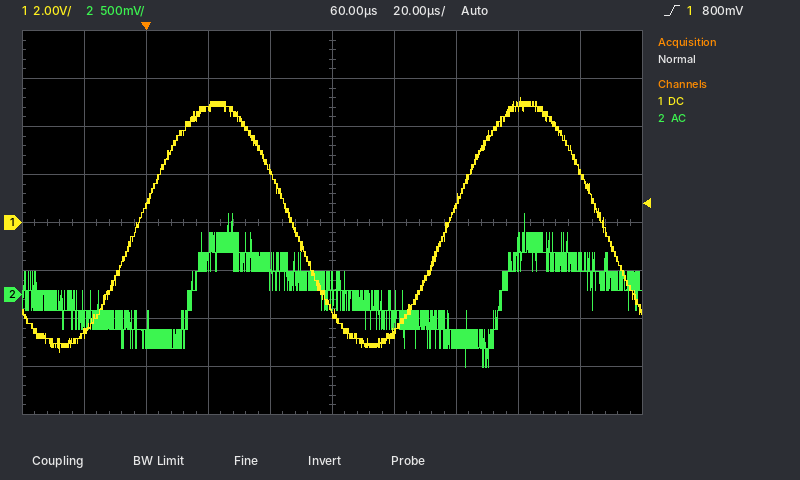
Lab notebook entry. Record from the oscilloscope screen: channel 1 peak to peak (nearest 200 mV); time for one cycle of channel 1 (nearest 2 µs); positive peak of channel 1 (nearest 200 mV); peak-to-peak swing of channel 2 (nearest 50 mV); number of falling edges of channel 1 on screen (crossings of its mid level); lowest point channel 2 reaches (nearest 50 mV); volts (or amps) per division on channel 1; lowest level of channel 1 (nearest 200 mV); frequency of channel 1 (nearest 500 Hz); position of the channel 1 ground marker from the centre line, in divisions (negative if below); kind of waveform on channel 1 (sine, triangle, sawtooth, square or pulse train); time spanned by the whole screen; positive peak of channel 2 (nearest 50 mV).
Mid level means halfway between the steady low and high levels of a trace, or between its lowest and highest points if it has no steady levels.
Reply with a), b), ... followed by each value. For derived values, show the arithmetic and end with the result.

a) 5.2 V − (-5.4 V) = 10.6 V
b) 100 µs
c) 5.2 V
d) 850 mV − (-750 mV) = 1.60 V
e) 2
f) -750 mV
g) 2 V
h) -5.4 V
i) 1 / 100 µs ≈ 10.0 kHz
j) 0.0 div
k) sine
l) 200 µs
m) 850 mV
